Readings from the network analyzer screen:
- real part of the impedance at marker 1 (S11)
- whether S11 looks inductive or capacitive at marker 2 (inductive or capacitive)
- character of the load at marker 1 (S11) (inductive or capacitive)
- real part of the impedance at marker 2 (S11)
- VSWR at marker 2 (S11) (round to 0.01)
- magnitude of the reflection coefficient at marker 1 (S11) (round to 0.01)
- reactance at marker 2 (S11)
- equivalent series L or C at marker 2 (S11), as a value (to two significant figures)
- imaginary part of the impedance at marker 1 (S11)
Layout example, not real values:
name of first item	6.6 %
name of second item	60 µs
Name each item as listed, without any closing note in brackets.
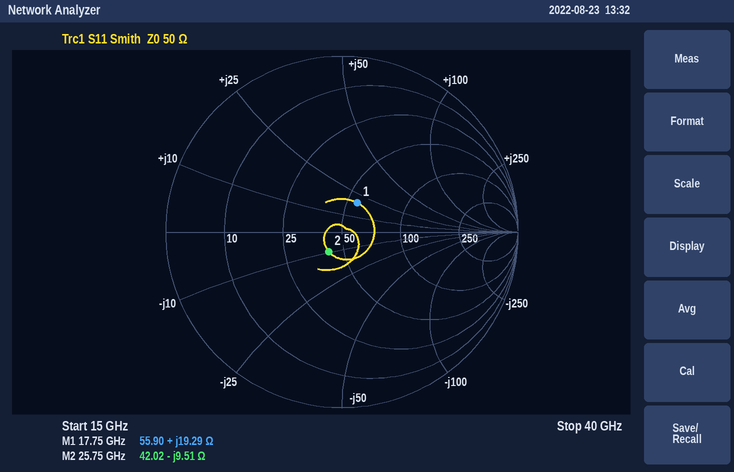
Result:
real part of the impedance at marker 1	55.90 Ω
whether S11 looks inductive or capacitive at marker 2	capacitive
character of the load at marker 1 (S11)	inductive
real part of the impedance at marker 2	42.02 Ω
VSWR at marker 2 (S11)	1.31
magnitude of the reflection coefficient at marker 1 (S11)	0.19
reactance at marker 2	-9.51 Ω
equivalent series L or C at marker 2 (S11), as a value	650 fF
imaginary part of the impedance at marker 1	+19.29 Ω
